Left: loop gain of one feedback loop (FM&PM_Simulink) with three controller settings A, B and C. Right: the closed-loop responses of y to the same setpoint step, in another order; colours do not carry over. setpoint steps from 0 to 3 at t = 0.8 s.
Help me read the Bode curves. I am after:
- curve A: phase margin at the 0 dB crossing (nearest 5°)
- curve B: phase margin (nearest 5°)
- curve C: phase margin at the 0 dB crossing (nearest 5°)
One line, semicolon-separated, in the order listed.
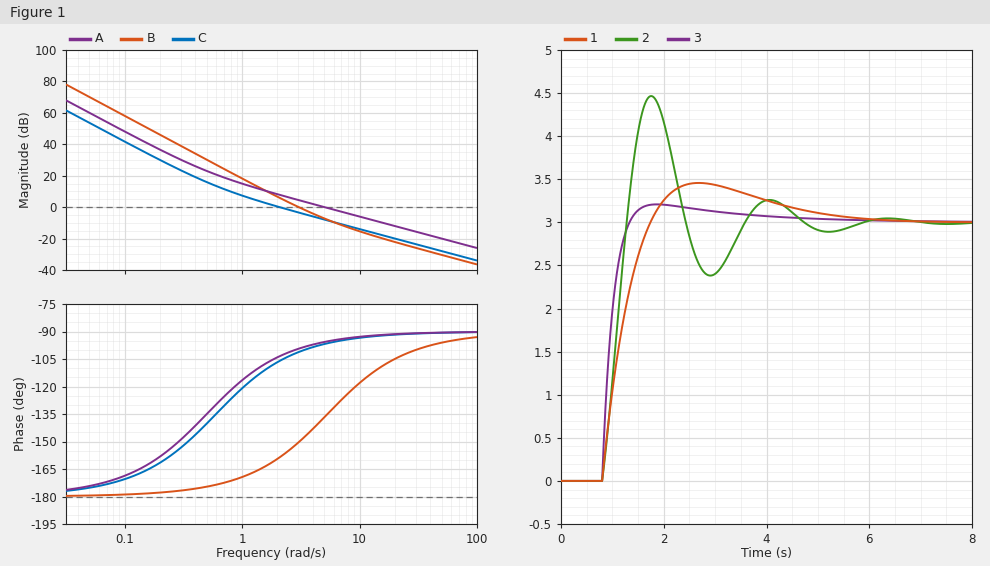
85°; 30°; 75°
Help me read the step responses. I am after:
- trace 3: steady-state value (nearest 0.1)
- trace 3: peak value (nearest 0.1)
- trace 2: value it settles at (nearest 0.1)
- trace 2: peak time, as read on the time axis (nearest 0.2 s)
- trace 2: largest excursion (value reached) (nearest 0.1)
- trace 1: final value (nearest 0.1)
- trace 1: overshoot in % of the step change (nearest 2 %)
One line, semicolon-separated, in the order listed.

3.0; 3.2; 3.0; 1.8 s; 4.5; 3.0; 16 %
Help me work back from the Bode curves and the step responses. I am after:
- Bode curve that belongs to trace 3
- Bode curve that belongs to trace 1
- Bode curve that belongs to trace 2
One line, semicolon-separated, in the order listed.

A; C; B
